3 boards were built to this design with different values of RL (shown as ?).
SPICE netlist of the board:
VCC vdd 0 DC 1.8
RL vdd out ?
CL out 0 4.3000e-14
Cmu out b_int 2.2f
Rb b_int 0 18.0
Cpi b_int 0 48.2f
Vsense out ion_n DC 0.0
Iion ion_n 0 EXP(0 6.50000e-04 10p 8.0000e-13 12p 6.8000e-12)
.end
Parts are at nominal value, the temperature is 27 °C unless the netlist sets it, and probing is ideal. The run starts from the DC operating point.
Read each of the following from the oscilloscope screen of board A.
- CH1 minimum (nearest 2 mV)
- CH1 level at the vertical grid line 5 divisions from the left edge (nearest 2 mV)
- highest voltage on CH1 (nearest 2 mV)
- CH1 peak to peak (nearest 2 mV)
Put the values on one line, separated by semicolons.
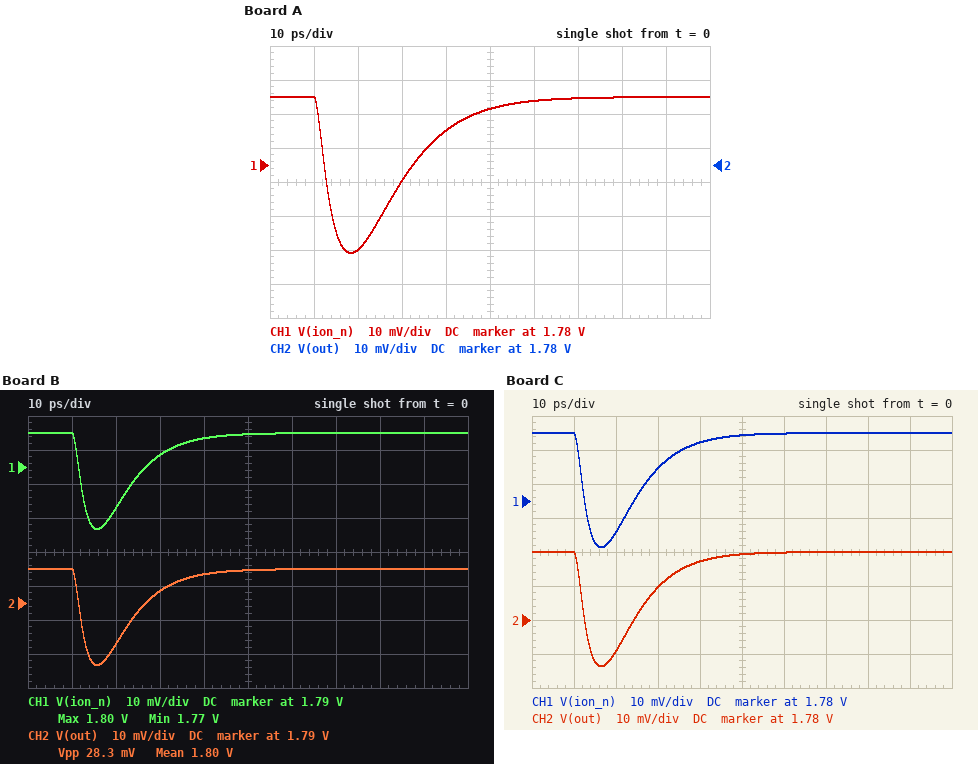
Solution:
1.754 V; 1.796 V; 1.800 V; 46 mV
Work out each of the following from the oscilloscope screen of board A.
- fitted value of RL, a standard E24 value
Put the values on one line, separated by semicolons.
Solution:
180 Ω
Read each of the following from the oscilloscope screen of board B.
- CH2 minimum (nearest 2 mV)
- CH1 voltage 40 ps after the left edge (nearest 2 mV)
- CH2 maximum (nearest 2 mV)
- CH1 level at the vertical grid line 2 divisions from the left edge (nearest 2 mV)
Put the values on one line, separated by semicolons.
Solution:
1.772 V; 1.798 V; 1.800 V; 1.778 V
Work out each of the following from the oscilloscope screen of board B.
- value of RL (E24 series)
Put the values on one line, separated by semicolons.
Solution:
75 Ω
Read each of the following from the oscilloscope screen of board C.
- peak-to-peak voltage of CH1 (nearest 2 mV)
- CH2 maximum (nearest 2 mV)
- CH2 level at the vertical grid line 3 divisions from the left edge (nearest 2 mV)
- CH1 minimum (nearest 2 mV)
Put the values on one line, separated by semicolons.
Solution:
34 mV; 1.800 V; 1.790 V; 1.766 V
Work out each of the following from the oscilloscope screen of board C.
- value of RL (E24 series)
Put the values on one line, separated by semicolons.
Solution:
100 Ω
